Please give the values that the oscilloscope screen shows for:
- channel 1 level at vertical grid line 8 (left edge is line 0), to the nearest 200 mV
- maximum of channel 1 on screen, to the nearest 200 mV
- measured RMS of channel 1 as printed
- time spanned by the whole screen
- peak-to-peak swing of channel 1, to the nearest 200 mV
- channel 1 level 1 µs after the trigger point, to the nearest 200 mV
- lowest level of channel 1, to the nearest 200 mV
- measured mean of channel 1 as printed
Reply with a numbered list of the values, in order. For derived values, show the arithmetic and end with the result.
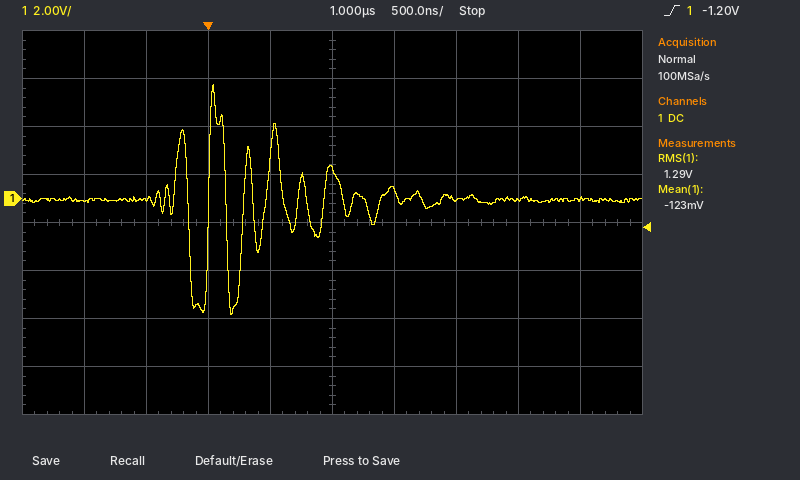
1. 0.0 V
2. 4.8 V
3. 1.29 V
4. 5 µs
5. 4.8 V − (-4.8 V) = 9.6 V
6. 1.2 V
7. -4.8 V
8. -123 mV
